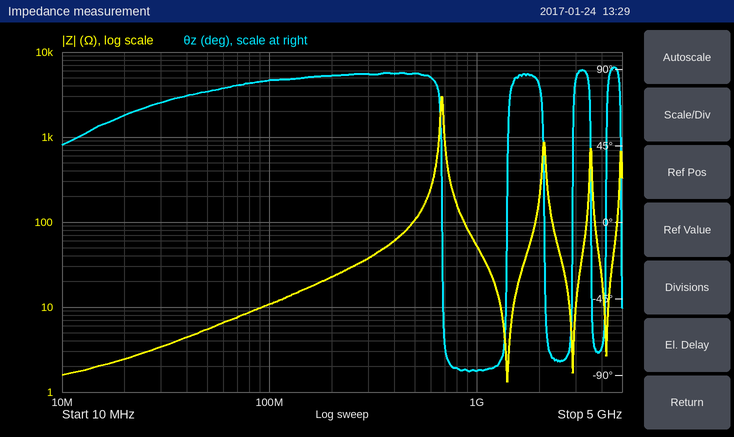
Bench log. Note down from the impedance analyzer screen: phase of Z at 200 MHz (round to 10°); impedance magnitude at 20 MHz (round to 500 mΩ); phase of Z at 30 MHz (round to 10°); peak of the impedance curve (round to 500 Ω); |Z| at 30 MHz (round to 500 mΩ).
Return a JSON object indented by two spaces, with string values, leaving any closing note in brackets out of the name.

{
  "phase of Z at 200 MHz": "90°",
  "impedance magnitude at 20 MHz": "2.5 Ω",
  "phase of Z at 30 MHz": "70°",
  "peak of the impedance curve": "3.0 kΩ",
  "|Z| at 30 MHz": "3.5 Ω"
}
